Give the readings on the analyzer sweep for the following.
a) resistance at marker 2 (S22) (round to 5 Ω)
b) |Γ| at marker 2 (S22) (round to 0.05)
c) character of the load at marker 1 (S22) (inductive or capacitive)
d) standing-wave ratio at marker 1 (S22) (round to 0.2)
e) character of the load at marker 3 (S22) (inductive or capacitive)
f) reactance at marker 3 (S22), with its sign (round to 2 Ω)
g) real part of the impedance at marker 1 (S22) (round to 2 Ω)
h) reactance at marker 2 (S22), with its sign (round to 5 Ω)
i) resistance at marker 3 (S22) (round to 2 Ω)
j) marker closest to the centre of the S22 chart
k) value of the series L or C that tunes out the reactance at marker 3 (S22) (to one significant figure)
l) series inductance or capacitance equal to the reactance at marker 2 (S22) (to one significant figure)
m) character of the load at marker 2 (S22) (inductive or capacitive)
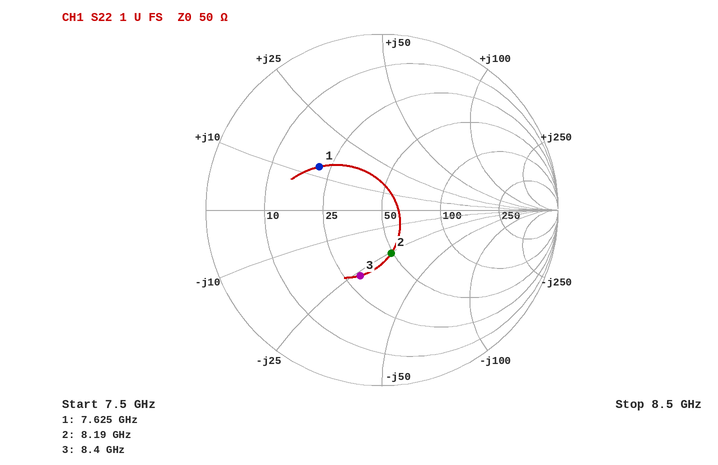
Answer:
50 Ω
0.25
inductive
2.6
capacitive
-26 Ω
22 Ω
-25 Ω
30 Ω
marker 2
500 pH
800 fF
capacitive
